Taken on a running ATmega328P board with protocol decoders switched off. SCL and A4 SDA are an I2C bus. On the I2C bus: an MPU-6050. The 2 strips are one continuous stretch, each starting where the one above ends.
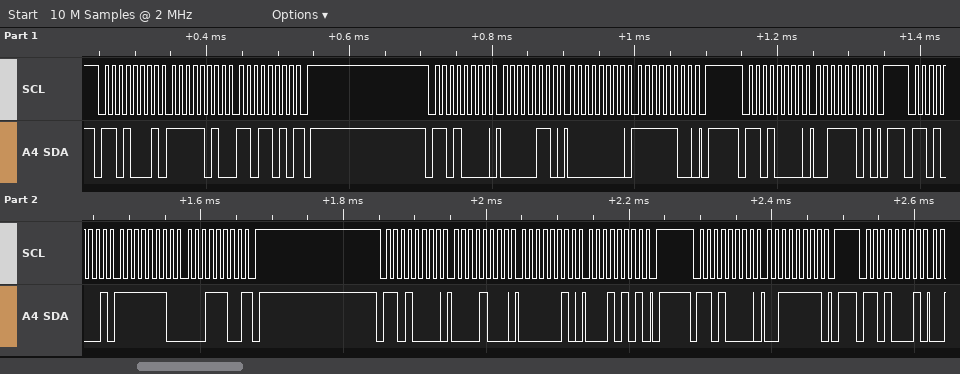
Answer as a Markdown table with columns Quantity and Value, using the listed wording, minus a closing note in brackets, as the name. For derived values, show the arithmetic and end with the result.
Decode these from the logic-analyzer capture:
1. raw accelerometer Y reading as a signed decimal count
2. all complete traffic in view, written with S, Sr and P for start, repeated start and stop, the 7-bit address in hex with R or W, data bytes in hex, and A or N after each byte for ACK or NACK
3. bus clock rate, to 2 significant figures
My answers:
| Quantity | Value |
|---|---|
| raw accelerometer Y reading as a signed decimal count | 0xFE1C = -484 |
| all complete traffic in view, written with S, Sr and P for start, repeated start and stop, the 7-bit address in hex with R or W, data bytes in hex, and A or N after each byte for ACK or NACK | S 68R A FA A DA N P S 68W A 06 A 00 A FC A P S 68W A 3D A P S 68R A FE A 1C N P S 68W A 08 A 02 A 15 A P S 68W A 3F A P S 68R A |
| bus clock rate, to 2 significant figures | 100 kHz |
